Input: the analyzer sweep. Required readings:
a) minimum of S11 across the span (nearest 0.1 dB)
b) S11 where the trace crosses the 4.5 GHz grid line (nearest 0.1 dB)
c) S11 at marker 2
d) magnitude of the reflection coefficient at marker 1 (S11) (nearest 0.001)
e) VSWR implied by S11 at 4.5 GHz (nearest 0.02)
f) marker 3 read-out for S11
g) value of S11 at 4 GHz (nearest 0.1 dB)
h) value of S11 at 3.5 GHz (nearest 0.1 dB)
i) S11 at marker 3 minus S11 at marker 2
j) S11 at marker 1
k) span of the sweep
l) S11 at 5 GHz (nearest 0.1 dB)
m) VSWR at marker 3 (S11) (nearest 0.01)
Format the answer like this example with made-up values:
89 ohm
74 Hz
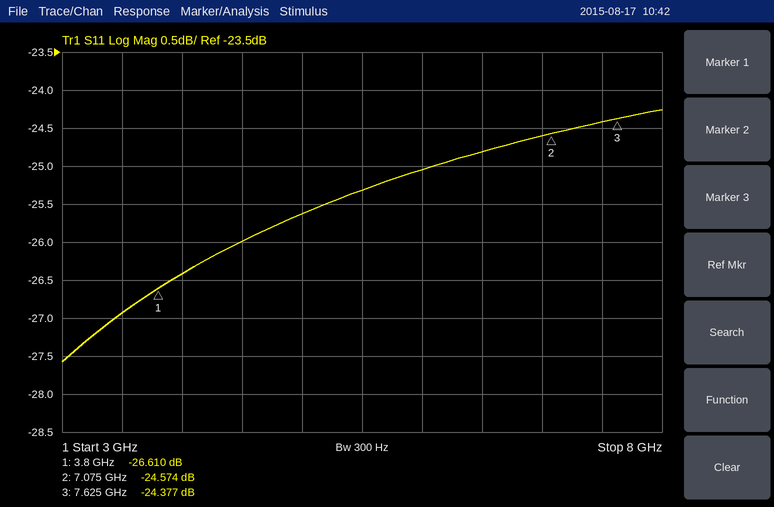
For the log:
-27.6 dB
-26.0 dB
-24.574 dB
0.047
1.10
-24.377 dB
-26.4 dB
-26.9 dB
0.197 dB
-26.610 dB
5 GHz
-25.6 dB
1.13
